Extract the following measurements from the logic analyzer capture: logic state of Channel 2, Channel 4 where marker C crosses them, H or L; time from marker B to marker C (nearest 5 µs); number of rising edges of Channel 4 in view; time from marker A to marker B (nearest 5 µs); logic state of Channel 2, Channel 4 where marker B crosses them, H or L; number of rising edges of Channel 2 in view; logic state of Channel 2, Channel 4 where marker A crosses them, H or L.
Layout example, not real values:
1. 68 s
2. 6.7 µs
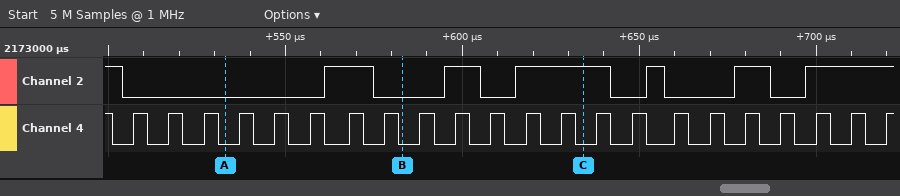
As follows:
1. Channel 2=H, Channel 4=L
2. 50 µs
3. 22
4. 50 µs
5. Channel 2=L, Channel 4=L
6. 6
7. Channel 2=L, Channel 4=L
